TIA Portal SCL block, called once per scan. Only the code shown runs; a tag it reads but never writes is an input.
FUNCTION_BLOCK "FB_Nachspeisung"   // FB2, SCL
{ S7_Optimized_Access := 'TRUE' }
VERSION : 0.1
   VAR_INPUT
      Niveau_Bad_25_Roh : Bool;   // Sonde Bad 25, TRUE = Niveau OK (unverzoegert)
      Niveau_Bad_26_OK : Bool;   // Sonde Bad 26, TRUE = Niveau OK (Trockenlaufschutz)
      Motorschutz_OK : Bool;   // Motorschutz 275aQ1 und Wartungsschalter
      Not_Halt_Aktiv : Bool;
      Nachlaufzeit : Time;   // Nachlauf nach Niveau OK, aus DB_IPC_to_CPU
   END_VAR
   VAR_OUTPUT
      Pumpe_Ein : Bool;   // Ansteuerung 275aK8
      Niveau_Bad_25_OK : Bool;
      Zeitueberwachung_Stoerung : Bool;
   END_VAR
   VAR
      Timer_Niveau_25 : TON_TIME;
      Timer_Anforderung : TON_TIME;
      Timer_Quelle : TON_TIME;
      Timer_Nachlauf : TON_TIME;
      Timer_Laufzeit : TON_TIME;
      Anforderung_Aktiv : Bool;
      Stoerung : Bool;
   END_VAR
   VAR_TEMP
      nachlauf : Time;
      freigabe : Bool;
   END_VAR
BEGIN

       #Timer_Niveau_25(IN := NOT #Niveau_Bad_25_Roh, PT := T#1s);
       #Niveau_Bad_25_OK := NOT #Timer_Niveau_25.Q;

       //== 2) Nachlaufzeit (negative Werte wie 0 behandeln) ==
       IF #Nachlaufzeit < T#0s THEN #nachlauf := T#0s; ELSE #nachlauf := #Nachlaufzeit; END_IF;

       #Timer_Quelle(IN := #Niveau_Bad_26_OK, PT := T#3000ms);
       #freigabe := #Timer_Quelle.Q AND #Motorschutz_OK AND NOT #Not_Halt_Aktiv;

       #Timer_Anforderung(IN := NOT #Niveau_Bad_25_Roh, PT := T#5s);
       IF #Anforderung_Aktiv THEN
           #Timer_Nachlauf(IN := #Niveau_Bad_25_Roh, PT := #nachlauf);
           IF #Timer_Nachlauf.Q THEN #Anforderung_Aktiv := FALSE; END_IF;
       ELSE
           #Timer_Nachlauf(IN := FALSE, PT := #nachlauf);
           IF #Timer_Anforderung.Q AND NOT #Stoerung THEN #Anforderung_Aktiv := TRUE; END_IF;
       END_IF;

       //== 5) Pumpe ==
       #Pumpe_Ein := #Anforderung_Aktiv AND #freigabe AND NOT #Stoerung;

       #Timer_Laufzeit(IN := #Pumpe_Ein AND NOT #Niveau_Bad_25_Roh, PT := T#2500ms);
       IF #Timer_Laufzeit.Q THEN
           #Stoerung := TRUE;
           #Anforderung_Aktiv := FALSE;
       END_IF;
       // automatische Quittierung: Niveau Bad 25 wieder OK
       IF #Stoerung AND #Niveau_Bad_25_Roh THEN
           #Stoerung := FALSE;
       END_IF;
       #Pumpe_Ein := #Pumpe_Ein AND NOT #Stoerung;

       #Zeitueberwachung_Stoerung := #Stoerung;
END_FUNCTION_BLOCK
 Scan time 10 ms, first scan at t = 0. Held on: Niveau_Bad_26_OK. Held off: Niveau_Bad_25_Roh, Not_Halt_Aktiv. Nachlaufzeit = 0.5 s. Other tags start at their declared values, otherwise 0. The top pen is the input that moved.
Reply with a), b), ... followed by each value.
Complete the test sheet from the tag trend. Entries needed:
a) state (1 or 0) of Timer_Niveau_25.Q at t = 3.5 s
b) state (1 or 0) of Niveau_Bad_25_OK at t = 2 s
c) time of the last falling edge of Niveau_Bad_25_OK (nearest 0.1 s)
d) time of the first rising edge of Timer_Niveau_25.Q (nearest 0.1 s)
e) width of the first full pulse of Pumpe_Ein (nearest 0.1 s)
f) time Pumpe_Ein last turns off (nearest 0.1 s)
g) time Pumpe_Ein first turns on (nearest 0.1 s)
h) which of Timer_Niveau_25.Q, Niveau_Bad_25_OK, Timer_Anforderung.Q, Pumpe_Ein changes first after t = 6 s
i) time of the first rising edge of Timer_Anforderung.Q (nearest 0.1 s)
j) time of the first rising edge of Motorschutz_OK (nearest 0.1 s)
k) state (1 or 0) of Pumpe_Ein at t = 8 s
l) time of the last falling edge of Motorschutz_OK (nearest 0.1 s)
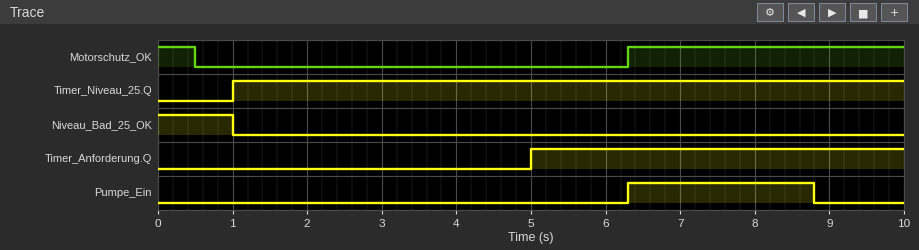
a) 1
b) 0
c) 1.0 s
d) 1.0 s
e) 2.5 s
f) 8.8 s
g) 6.3 s
h) Pumpe_Ein
i) 5.0 s
j) 6.3 s
k) 1
l) 0.5 s
